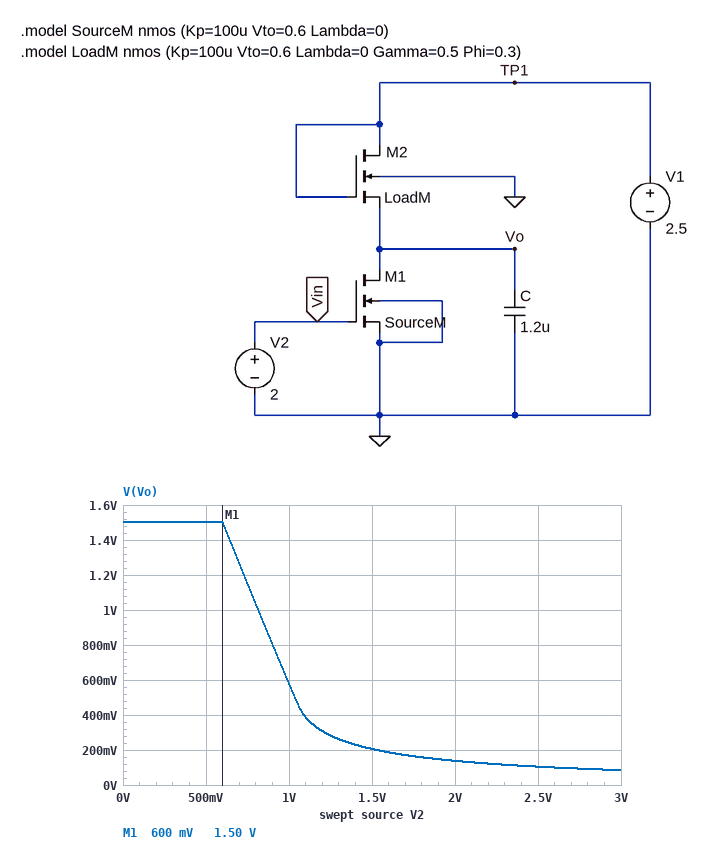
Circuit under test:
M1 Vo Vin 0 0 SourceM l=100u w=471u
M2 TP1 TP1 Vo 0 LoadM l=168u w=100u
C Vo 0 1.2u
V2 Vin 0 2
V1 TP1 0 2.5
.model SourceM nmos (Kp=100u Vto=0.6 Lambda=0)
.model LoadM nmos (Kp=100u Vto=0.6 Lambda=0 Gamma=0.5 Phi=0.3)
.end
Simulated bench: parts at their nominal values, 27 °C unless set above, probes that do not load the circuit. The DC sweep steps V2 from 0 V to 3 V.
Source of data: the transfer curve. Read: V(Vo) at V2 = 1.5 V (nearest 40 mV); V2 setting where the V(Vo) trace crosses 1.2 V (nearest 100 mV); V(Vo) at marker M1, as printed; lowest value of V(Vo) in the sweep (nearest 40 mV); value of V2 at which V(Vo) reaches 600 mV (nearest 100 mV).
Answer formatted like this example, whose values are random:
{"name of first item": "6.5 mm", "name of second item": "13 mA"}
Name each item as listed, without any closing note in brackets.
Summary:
{"V(Vo) at V2 = 1.5 V": "200 mV", "V2 setting where the V(Vo) trace crosses 1.2 V": "700 mV", "V(Vo) at marker M1, as printed": "1.50 V", "lowest value of V(Vo) in the sweep": "80 mV", "value of V2 at which V(Vo) reaches 600 mV": "1.0 V"}
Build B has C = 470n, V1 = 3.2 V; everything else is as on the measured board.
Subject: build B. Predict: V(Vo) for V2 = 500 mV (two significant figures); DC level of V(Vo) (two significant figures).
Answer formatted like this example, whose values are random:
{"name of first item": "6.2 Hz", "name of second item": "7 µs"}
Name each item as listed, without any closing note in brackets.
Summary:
{"V(Vo) for V2 = 500 mV": "2.1 V", "DC level of V(Vo)": "250 mV"}
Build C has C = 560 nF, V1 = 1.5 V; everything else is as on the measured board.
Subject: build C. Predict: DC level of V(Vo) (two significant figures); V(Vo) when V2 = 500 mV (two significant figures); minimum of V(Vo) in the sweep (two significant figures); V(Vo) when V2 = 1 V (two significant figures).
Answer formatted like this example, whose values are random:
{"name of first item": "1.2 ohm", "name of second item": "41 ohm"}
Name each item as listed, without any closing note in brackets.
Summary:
{"DC level of V(Vo)": "33 mV", "V(Vo) when V2 = 500 mV": "680 mV", "minimum of V(Vo) in the sweep": "20 mV", "V(Vo) when V2 = 1 V": "100 mV"}
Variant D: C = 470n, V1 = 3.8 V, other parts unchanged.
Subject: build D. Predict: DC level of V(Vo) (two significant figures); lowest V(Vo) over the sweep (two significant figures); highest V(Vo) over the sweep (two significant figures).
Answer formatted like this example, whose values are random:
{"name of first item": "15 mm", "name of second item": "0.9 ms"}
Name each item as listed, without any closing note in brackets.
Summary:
{"DC level of V(Vo)": "380 mV", "lowest V(Vo) over the sweep": "230 mV", "highest V(Vo) over the sweep": "2.6 V"}
